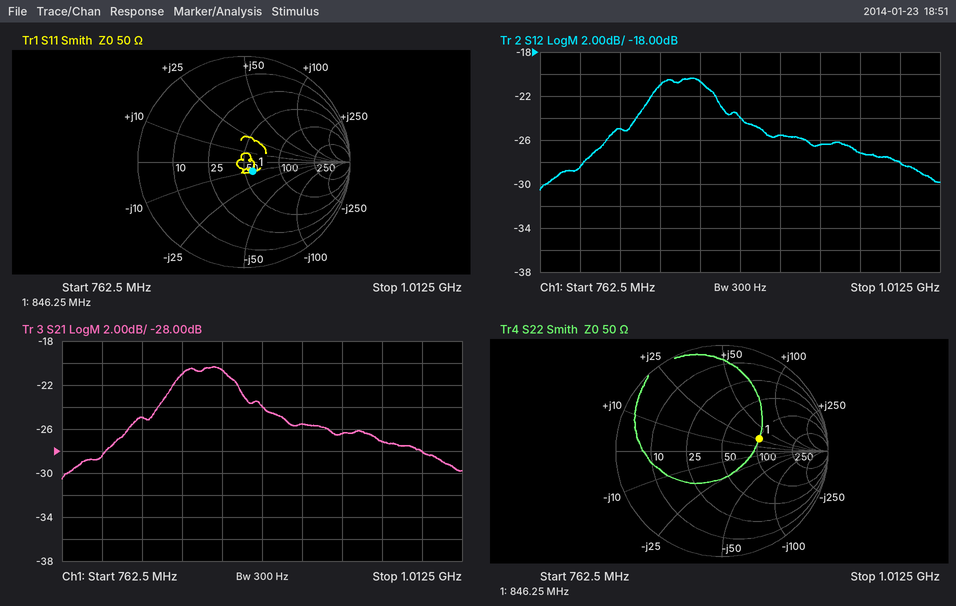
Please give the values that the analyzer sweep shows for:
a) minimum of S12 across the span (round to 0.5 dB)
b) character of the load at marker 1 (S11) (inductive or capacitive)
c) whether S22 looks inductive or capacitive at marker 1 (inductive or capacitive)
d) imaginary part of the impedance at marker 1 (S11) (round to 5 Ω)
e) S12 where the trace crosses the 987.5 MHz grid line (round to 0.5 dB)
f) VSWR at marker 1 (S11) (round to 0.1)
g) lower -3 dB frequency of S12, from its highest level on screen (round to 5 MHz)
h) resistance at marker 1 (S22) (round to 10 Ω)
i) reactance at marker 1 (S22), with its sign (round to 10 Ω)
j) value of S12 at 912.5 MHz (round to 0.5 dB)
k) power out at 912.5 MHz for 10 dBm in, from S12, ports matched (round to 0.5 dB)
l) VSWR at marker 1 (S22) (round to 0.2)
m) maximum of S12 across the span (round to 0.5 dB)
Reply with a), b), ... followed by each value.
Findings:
a) -30.5 dB
b) capacitive
c) inductive
d) -10 Ω
e) -28.0 dB
f) 1.3
g) 825 MHz
h) 100 Ω
i) +30 Ω
j) -25.5 dB
k) -15.5 dBm
l) 2.2
m) -20.5 dB
